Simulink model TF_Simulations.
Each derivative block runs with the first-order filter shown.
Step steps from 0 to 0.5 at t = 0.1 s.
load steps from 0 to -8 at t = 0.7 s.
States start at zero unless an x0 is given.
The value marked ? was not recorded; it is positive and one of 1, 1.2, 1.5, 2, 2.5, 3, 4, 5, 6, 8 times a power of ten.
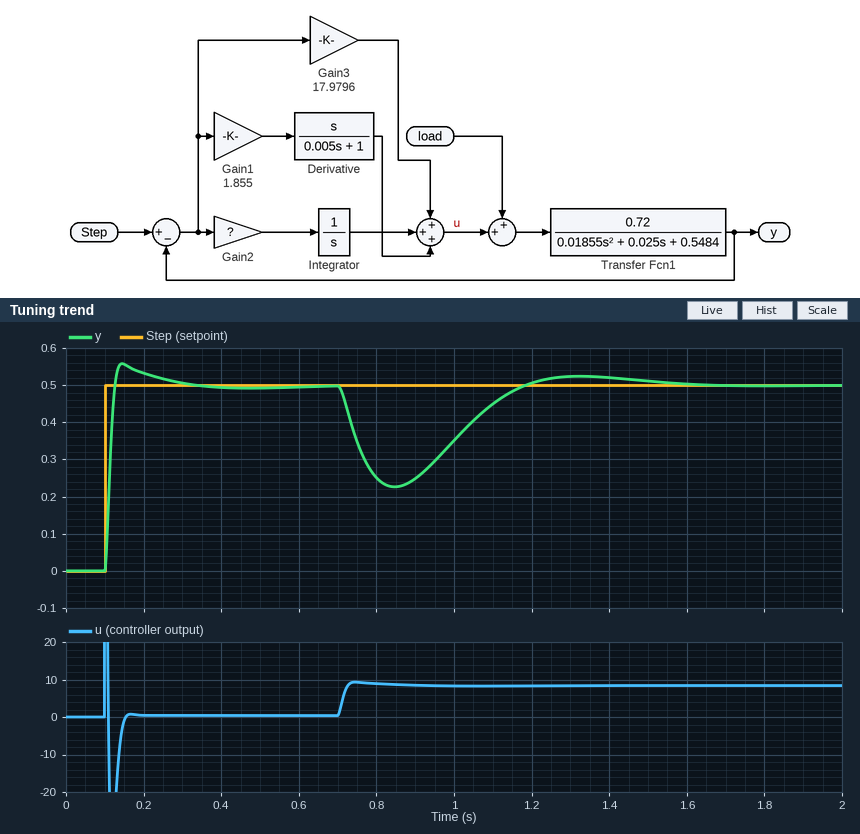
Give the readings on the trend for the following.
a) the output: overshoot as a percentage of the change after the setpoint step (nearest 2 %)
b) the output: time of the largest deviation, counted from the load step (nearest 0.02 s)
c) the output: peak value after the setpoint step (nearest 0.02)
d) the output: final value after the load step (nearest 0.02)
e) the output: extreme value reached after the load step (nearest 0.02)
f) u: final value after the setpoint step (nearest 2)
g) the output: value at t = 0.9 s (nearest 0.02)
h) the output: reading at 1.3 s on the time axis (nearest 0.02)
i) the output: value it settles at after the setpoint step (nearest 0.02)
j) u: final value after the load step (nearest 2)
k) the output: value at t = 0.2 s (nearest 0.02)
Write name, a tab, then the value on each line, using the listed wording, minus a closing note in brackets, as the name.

the output: overshoot as a percentage of the change after the setpoint step	12 %
the output: time of the largest deviation, counted from the load step	0.14 s
the output: peak value after the setpoint step	0.56
the output: final value after the load step	0.50
the output: extreme value reached after the load step	0.22
u: final value after the setpoint step	0
the output: value at t = 0.9 s	0.24
the output: reading at 1.3 s on the time axis	0.52
the output: value it settles at after the setpoint step	0.50
u: final value after the load step	8
the output: value at t = 0.2 s	0.54
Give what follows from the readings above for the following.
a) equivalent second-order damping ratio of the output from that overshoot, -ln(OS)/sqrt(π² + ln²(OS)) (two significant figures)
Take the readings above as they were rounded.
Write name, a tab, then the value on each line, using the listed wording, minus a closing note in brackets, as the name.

equivalent second-order damping ratio of the output from that overshoot, -ln(OS)/sqrt(π² + ln²(OS))	0.56
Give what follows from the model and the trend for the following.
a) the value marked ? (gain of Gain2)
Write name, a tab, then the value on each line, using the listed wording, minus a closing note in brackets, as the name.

the value marked ?	120
